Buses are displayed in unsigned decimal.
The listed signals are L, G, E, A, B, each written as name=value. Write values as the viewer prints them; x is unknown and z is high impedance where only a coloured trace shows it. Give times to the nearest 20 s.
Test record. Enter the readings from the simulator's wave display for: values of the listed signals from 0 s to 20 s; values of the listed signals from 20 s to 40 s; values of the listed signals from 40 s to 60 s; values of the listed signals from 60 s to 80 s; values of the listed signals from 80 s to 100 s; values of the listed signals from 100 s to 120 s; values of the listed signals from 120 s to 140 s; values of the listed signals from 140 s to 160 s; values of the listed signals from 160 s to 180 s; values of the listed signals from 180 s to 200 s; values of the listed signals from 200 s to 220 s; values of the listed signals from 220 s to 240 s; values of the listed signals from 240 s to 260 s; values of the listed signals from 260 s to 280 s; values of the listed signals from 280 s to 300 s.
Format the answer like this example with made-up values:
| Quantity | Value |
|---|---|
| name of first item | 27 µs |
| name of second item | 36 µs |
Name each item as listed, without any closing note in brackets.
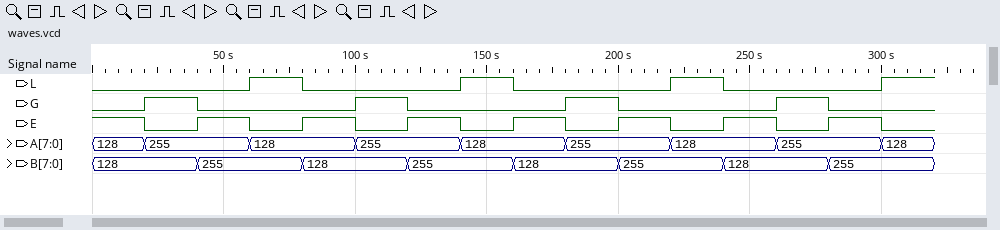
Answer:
| Quantity | Value |
|---|---|
| values of the listed signals from 0 s to 20 s | L=0, G=0, E=1, A=128, B=128 |
| values of the listed signals from 20 s to 40 s | L=0, G=1, E=0, A=255, B=128 |
| values of the listed signals from 40 s to 60 s | L=0, G=0, E=1, A=255, B=255 |
| values of the listed signals from 60 s to 80 s | L=1, G=0, E=0, A=128, B=255 |
| values of the listed signals from 80 s to 100 s | L=0, G=0, E=1, A=128, B=128 |
| values of the listed signals from 100 s to 120 s | L=0, G=1, E=0, A=255, B=128 |
| values of the listed signals from 120 s to 140 s | L=0, G=0, E=1, A=255, B=255 |
| values of the listed signals from 140 s to 160 s | L=1, G=0, E=0, A=128, B=255 |
| values of the listed signals from 160 s to 180 s | L=0, G=0, E=1, A=128, B=128 |
| values of the listed signals from 180 s to 200 s | L=0, G=1, E=0, A=255, B=128 |
| values of the listed signals from 200 s to 220 s | L=0, G=0, E=1, A=255, B=255 |
| values of the listed signals from 220 s to 240 s | L=1, G=0, E=0, A=128, B=255 |
| values of the listed signals from 240 s to 260 s | L=0, G=0, E=1, A=128, B=128 |
| values of the listed signals from 260 s to 280 s | L=0, G=1, E=0, A=255, B=128 |
| values of the listed signals from 280 s to 300 s | L=0, G=0, E=1, A=255, B=255 |
